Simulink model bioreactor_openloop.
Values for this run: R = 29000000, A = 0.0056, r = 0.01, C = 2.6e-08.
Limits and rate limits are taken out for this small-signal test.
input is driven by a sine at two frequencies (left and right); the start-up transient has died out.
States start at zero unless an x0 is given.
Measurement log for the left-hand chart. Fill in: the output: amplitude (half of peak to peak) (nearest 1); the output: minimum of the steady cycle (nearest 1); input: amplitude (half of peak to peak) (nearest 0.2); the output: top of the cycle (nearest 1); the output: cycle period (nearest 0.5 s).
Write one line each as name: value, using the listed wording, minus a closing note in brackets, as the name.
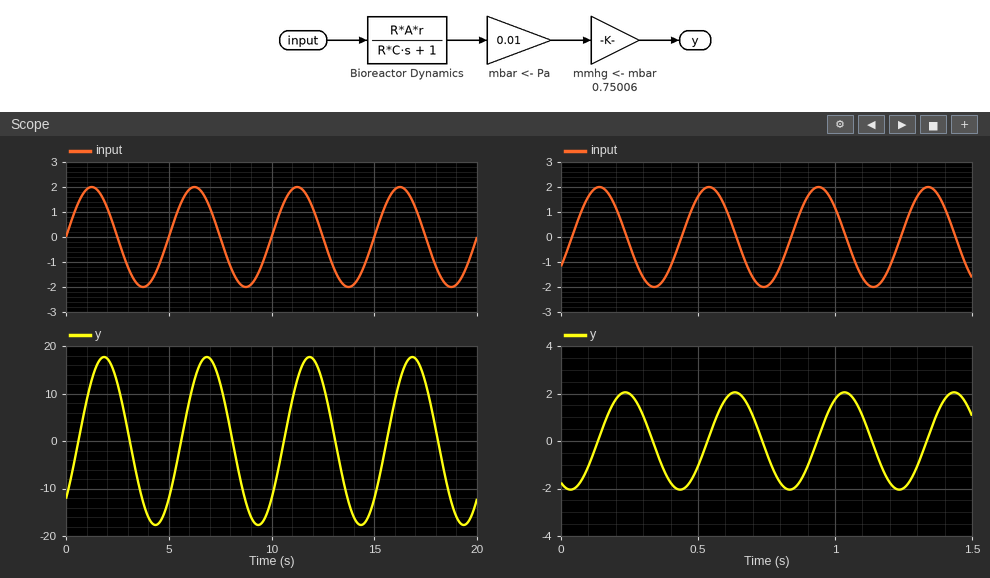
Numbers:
the output: amplitude (half of peak to peak): 18
the output: minimum of the steady cycle: -18
input: amplitude (half of peak to peak): 2.0
the output: top of the cycle: 18
the output: cycle period: 5.0 s
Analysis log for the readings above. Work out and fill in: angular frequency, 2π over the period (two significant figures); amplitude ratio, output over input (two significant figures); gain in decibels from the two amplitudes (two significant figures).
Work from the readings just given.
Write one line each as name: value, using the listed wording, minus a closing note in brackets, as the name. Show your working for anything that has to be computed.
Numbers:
angular frequency, 2π over the period: 2π / 5 = 1.3 rad/s
amplitude ratio, output over input: 18 / 2 = 9.0
gain in decibels from the two amplitudes: 20 log10(18 / 2) = 19 dB
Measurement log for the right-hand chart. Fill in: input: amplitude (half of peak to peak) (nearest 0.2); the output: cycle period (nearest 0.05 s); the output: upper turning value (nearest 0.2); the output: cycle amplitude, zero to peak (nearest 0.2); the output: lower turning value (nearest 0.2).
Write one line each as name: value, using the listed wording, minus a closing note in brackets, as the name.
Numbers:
input: amplitude (half of peak to peak): 2.0
the output: cycle period: 0.40 s
the output: upper turning value: 2.0
the output: cycle amplitude, zero to peak: 2.0
the output: lower turning value: -2.0
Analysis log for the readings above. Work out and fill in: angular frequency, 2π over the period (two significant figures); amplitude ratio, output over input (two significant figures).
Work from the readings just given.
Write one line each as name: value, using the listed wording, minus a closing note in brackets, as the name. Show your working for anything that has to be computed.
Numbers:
angular frequency, 2π over the period: 2π / 0.4 = 16 rad/s
amplitude ratio, output over input: 2 / 2 = 1.0
